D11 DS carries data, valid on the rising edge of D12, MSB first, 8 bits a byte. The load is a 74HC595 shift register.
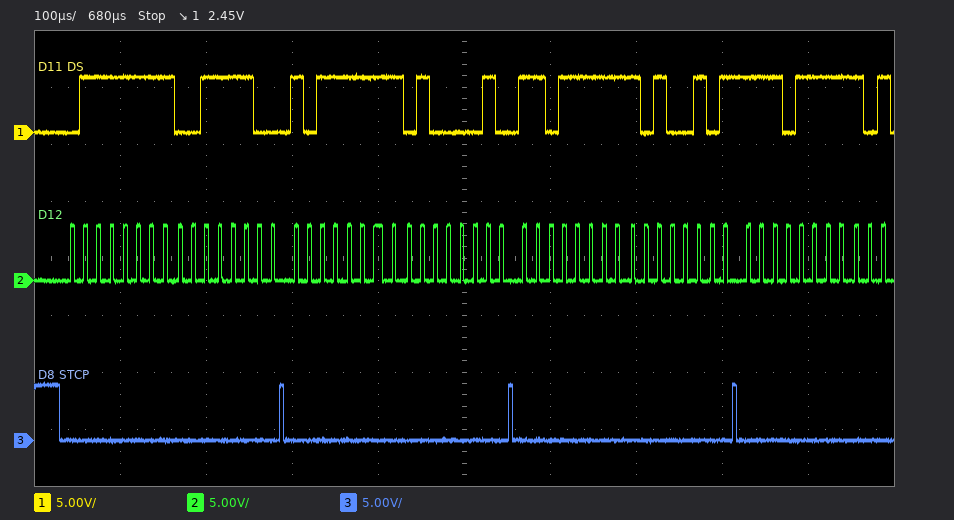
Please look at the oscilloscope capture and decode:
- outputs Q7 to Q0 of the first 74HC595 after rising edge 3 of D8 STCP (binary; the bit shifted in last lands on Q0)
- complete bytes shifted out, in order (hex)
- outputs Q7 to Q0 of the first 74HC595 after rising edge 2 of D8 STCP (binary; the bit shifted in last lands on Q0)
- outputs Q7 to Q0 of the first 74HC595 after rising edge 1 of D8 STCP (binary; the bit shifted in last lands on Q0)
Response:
10100101
7F 3C BF 42 DF A5 EF
01000010
00111100
